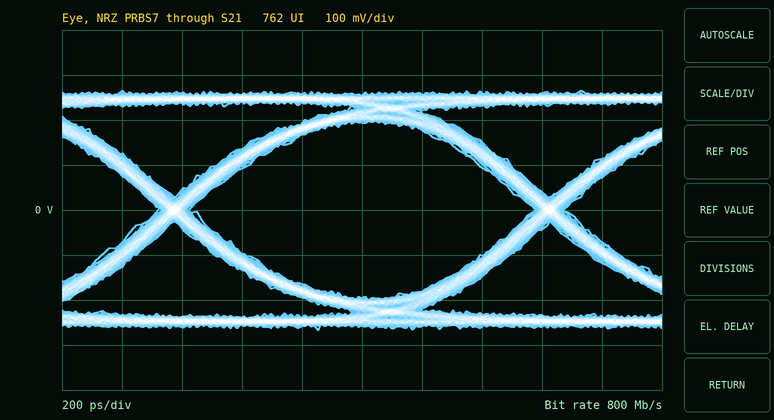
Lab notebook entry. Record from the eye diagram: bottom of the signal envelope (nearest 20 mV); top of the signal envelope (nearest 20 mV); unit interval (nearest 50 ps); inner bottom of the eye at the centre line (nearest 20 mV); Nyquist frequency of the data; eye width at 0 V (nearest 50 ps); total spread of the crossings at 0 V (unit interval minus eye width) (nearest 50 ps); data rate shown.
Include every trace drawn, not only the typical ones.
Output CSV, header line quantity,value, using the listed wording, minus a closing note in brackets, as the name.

quantity,value
bottom of the signal envelope,-260 mV
top of the signal envelope,260 mV
unit interval,1.25 ns
inner bottom of the eye at the centre line,-200 mV
Nyquist frequency of the data,400 MHz
eye width at 0 V,1.15 ns
total spread of the crossings at 0 V (unit interval minus eye width),100 ps
data rate shown,800 Mb/s
